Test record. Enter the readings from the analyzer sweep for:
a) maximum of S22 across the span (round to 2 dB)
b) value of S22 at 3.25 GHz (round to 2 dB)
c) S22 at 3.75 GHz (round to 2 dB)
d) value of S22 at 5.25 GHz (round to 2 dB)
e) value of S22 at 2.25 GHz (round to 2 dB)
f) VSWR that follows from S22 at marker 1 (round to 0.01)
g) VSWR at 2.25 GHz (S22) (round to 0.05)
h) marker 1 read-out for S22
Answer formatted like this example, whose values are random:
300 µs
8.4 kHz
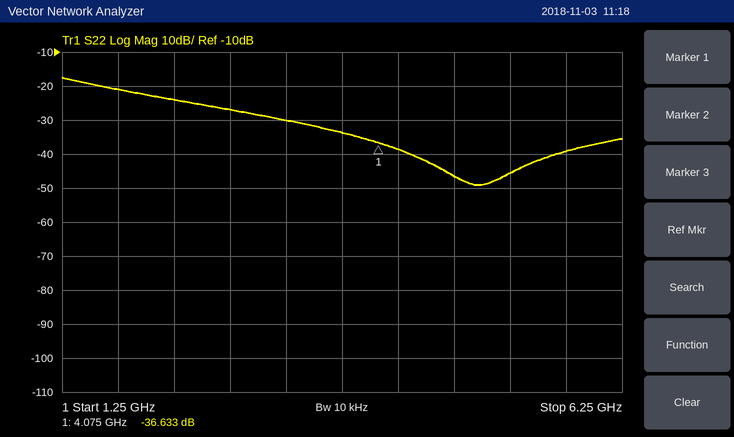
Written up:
-18 dB
-30 dB
-34 dB
-46 dB
-24 dB
1.03
1.15
-36.633 dB
